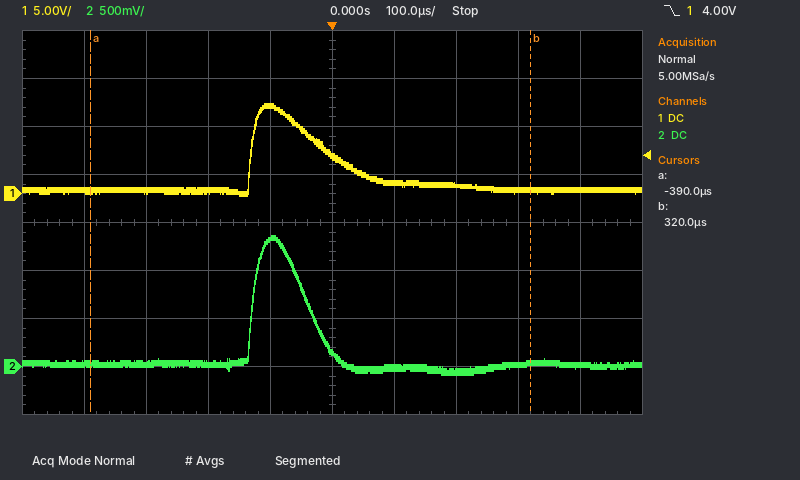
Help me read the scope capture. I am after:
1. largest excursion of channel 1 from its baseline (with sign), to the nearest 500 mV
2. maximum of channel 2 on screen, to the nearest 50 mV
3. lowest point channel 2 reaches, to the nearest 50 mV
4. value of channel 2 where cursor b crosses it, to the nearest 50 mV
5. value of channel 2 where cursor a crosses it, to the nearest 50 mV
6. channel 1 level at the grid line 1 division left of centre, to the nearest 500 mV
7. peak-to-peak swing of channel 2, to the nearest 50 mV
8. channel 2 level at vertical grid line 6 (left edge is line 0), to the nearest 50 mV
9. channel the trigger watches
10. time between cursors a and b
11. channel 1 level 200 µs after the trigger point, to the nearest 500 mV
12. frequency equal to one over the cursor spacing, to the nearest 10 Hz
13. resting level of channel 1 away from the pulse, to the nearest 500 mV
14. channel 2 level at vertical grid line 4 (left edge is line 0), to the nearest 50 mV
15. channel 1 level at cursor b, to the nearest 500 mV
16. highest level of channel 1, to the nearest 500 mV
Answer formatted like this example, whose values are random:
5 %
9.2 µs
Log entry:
+9.0 V
1.35 V
-100 mV
50 mV
50 mV
9.0 V
1.45 V
0 mV
channel 1
710 µs
1.0 V
1.41 kHz
500 mV
1.30 V
500 mV
9.5 V
